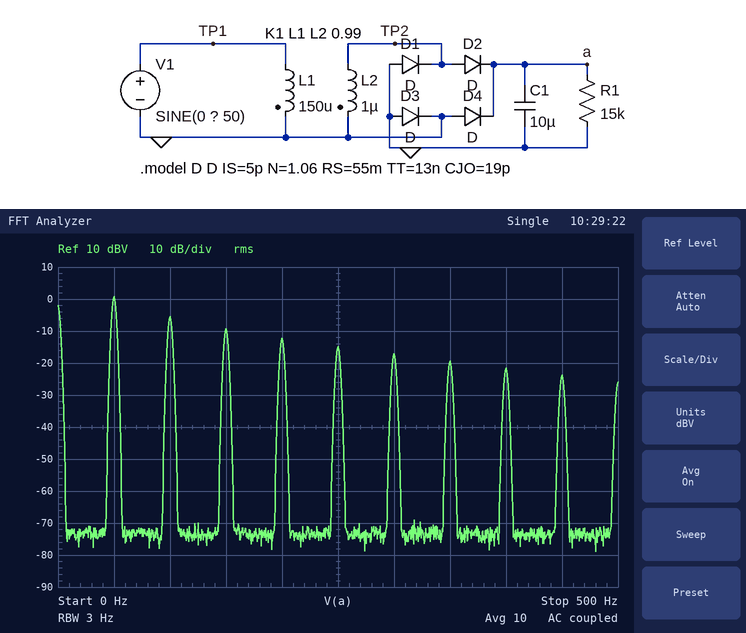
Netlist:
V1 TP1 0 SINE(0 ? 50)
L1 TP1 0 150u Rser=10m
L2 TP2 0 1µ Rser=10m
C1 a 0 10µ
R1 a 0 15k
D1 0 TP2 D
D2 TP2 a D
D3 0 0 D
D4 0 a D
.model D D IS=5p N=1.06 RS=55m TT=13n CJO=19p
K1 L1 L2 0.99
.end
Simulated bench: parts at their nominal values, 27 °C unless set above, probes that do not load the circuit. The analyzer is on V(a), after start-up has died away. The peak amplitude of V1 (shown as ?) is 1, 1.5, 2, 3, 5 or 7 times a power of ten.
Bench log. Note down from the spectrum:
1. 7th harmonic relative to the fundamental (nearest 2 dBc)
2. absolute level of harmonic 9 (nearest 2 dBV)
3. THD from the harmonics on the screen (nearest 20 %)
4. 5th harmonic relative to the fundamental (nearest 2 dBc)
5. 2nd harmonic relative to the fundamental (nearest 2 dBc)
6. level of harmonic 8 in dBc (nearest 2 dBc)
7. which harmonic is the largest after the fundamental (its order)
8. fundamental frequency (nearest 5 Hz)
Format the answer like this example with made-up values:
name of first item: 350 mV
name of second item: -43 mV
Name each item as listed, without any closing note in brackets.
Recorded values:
7th harmonic relative to the fundamental: -20 dBc
absolute level of harmonic 9: -24 dBV
THD from the harmonics on the screen: 60 %
5th harmonic relative to the fundamental: -16 dBc
2nd harmonic relative to the fundamental: -6 dBc
level of harmonic 8 in dBc: -22 dBc
which harmonic is the largest after the fundamental: 2
fundamental frequency: 50 Hz
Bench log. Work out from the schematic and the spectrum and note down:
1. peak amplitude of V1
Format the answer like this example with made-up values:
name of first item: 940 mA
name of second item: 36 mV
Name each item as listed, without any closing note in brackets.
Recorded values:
peak amplitude of V1: 500 V
